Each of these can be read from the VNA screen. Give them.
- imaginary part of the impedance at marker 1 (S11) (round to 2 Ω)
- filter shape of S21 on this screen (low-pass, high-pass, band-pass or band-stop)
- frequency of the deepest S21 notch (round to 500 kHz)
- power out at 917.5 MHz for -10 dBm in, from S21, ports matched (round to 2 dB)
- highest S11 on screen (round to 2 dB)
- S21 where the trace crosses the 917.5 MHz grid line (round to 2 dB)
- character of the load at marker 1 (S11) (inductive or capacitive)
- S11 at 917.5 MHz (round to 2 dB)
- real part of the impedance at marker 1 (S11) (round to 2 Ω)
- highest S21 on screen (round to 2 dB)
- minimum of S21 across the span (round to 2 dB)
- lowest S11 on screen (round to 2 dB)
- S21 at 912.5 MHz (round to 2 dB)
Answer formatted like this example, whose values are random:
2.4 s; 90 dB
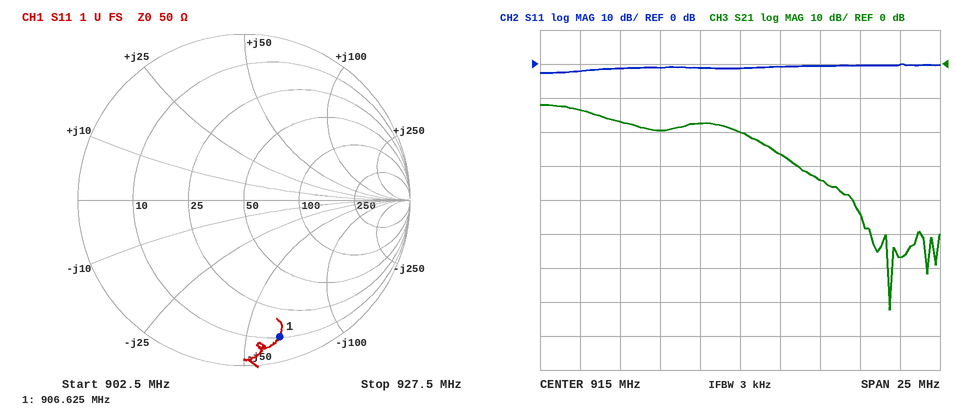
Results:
-64 Ω; low-pass; 924.5 MHz; -36 dBm; 0 dB; -26 dB; capacitive; 0 dB; 10 Ω; -12 dB; -72 dB; -2 dB; -18 dB
